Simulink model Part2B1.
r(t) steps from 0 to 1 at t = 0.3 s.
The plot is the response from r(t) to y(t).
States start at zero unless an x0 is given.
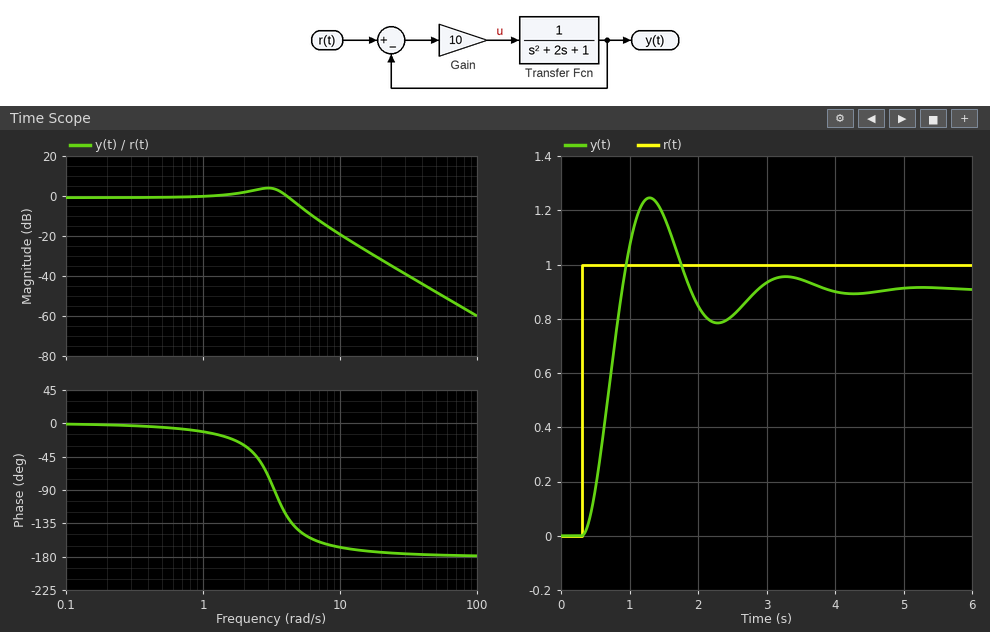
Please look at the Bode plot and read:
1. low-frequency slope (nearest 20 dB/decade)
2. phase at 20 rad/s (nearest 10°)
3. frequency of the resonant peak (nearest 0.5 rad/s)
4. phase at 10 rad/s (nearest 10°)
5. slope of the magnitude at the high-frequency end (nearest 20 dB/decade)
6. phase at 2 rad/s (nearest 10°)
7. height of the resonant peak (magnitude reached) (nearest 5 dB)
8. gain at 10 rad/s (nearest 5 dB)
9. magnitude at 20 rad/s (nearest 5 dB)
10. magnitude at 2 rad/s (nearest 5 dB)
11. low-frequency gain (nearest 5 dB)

0 dB/decade
-170°
3.0 rad/s
-170°
-40 dB/decade
-30°
5 dB
-20 dB
-30 dB
0 dB
0 dB
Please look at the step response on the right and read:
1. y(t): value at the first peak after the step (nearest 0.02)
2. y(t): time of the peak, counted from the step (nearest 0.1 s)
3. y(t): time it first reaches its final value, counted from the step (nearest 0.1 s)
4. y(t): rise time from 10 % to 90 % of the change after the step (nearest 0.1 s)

1.24
1.0 s
0.6 s
0.4 s
